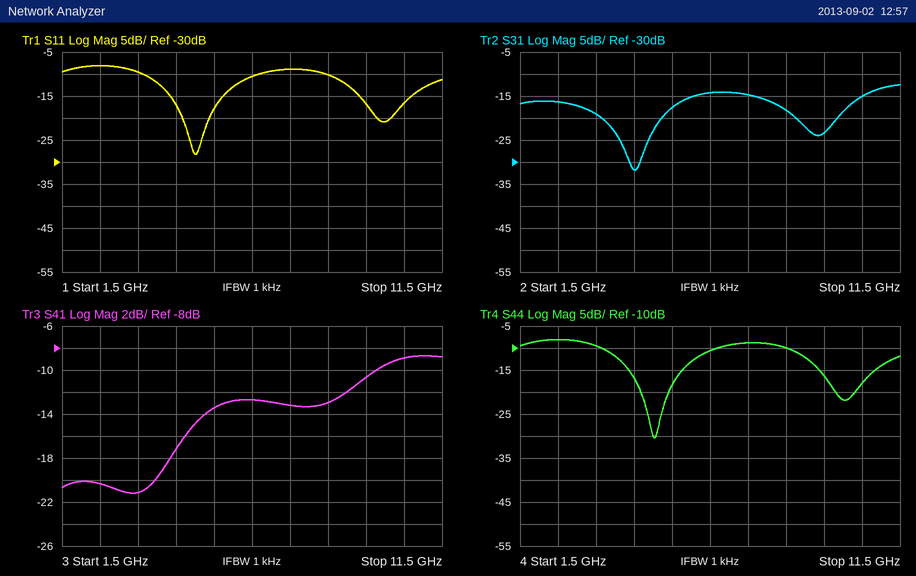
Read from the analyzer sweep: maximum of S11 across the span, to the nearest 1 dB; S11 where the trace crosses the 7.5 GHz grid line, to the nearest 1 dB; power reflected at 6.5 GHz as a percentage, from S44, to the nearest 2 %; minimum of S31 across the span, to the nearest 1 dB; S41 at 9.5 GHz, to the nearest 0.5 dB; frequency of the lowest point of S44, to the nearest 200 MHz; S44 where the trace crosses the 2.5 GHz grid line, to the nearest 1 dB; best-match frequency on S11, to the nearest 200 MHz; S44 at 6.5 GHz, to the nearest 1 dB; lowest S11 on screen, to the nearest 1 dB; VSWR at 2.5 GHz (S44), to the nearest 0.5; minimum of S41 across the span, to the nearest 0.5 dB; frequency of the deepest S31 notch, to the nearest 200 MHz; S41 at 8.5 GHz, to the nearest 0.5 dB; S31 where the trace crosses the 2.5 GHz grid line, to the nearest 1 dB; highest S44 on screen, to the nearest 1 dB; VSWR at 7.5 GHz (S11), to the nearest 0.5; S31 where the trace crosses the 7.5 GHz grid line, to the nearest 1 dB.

-8 dB
-9 dB
8 %
-32 dB
-10.5 dB
5.0 GHz
-8 dB
5.0 GHz
-11 dB
-28 dB
2.5
-21.0 dB
4.6 GHz
-13.0 dB
-16 dB
-8 dB
2.0
-15 dB
